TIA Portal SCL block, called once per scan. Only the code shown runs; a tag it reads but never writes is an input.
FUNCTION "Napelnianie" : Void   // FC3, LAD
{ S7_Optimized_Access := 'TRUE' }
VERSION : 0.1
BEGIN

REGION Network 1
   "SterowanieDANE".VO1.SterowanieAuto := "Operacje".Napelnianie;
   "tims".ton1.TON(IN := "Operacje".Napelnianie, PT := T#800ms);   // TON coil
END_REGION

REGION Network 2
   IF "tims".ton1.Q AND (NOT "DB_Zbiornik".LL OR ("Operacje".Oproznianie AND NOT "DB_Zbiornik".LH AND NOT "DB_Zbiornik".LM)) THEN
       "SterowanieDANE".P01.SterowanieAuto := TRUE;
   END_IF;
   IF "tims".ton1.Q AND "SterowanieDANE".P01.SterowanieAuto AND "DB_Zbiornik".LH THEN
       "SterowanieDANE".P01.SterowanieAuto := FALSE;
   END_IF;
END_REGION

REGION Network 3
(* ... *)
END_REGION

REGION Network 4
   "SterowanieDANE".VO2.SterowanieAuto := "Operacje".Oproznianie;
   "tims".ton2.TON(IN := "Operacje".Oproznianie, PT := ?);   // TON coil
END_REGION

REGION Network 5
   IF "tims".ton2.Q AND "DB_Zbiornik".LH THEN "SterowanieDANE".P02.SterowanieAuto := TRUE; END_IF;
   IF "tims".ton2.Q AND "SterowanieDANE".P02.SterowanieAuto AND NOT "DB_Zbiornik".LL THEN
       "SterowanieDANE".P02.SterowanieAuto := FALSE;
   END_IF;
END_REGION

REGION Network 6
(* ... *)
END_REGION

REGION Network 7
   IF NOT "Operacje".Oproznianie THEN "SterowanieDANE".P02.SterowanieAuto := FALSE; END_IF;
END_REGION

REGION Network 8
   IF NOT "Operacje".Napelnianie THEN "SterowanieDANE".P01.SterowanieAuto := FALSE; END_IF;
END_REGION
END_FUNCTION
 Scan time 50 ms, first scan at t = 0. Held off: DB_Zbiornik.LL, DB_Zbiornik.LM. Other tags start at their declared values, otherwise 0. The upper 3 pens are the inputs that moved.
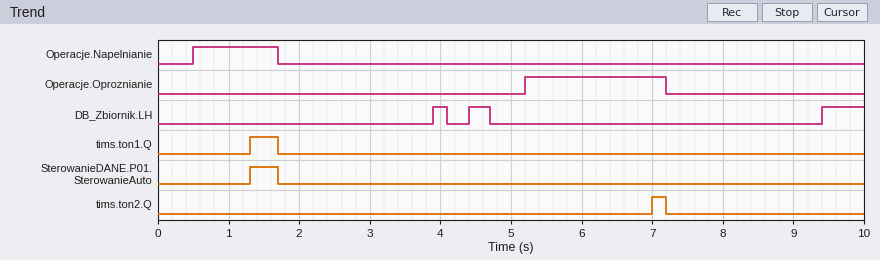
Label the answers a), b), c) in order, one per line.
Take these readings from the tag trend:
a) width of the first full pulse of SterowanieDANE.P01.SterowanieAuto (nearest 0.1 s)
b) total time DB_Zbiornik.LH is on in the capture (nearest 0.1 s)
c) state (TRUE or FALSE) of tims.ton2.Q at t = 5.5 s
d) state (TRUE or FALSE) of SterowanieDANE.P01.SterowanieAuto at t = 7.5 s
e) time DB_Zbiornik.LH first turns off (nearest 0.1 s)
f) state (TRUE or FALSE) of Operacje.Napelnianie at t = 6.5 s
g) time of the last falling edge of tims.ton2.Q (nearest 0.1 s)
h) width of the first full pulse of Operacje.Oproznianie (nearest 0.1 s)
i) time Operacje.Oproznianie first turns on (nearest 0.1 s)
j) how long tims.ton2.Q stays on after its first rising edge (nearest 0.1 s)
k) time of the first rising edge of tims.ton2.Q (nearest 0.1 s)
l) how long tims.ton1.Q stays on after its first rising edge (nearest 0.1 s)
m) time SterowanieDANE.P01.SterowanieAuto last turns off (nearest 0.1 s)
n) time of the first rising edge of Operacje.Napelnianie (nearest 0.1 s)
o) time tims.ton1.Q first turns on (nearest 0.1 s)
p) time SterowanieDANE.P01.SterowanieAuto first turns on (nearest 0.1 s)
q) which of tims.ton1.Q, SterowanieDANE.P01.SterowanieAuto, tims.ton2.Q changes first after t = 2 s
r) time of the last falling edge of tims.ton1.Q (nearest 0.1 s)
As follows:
a) 0.4 s
b) 1.1 s
c) FALSE
d) FALSE
e) 4.1 s
f) FALSE
g) 7.2 s
h) 2.0 s
i) 5.2 s
j) 0.2 s
k) 7.0 s
l) 0.4 s
m) 1.7 s
n) 0.5 s
o) 1.3 s
p) 1.3 s
q) tims.ton2.Q
r) 1.7 s
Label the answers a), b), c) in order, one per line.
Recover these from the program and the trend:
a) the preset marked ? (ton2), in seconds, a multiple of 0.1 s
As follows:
a) 1.8 s
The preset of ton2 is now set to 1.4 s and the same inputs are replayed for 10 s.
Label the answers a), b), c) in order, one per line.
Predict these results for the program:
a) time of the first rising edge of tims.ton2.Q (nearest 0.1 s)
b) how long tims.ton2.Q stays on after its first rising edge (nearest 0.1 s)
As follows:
a) 6.6 s
b) 0.6 s
